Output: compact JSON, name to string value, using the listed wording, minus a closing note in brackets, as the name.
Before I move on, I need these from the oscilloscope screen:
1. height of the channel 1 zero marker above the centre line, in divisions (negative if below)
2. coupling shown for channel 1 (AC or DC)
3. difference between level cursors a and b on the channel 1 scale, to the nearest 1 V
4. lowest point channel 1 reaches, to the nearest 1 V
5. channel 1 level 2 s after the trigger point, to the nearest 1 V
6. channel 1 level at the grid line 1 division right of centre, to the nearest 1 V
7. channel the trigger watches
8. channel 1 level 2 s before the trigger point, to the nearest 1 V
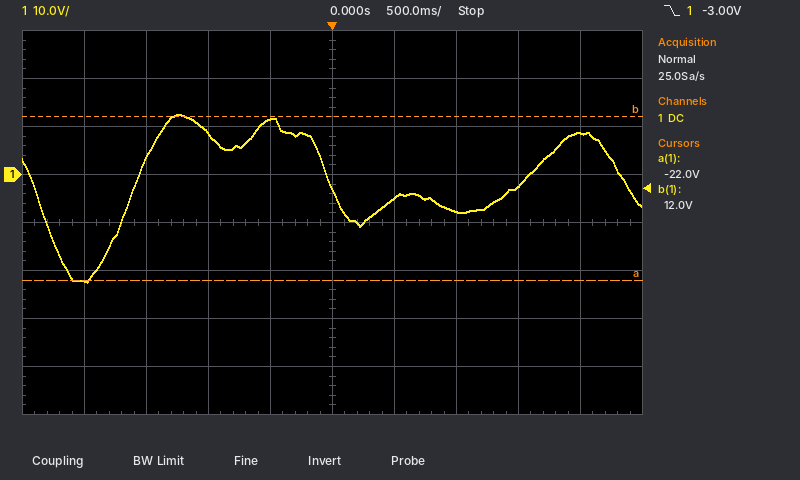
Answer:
{"height of the channel 1 zero marker above the centre line, in divisions": "+1.0 div", "coupling shown for channel 1": "DC", "difference between level cursors a and b on the channel 1 scale, to the nearest 1 V": "34 V", "lowest point channel 1 reaches, to the nearest 1 V": "-22 V", "channel 1 level 2 s after the trigger point, to the nearest 1 V": "9 V", "channel 1 level at the grid line 1 division right of centre, to the nearest 1 V": "-5 V", "channel the trigger watches": "channel 1", "channel 1 level 2 s before the trigger point, to the nearest 1 V": "-22 V"}
